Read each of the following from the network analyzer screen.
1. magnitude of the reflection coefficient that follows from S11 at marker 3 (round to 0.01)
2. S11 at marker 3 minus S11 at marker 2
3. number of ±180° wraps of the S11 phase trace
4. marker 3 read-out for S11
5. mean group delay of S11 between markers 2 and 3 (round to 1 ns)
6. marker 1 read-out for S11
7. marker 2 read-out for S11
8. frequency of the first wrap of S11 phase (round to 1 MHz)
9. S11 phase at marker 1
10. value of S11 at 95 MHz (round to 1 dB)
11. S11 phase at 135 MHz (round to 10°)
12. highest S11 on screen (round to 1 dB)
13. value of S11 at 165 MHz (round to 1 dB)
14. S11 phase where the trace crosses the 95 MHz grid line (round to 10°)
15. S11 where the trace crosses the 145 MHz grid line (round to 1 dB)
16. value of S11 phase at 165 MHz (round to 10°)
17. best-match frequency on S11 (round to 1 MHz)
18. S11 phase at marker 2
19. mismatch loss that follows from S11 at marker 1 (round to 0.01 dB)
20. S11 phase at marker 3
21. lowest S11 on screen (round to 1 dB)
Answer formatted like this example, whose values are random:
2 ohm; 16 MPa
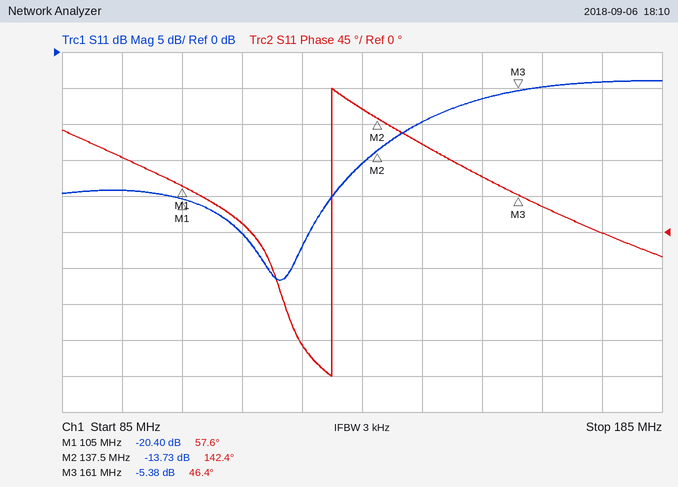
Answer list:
0.54; 8.35 dB; 1; -5.38 dB; 11 ns; -20.40 dB; -13.73 dB; 130 MHz; 57.6°; -19 dB; 150°; -4 dB; -5 dB; 90°; -10 dB; 30°; 121 MHz; 142.4°; 0.04 dB; 46.4°; -32 dB
